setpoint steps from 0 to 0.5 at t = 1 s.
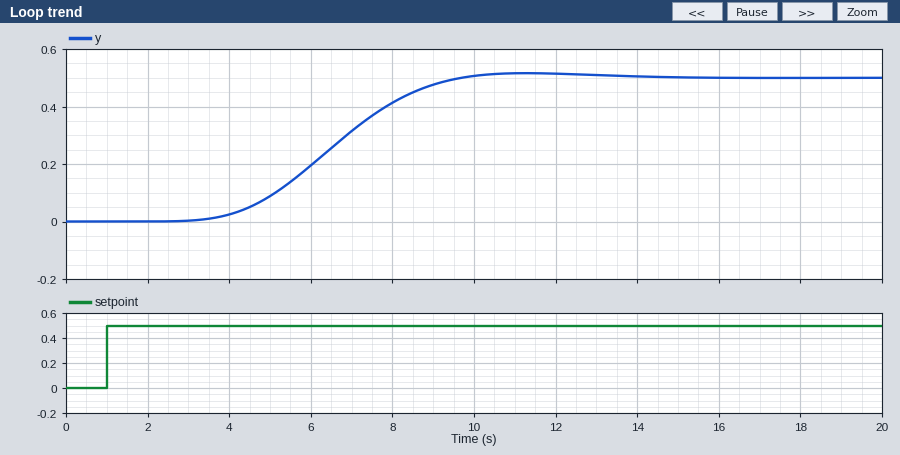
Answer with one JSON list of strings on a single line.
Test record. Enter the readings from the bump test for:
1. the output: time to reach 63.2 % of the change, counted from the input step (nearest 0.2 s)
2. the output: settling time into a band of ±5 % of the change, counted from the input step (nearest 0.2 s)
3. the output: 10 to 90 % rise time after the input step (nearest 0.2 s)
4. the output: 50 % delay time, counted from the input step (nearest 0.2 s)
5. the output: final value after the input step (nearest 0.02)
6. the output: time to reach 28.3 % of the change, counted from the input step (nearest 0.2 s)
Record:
["6.0 s", "8.0 s", "4.0 s", "5.4 s", "0.50", "4.6 s"]
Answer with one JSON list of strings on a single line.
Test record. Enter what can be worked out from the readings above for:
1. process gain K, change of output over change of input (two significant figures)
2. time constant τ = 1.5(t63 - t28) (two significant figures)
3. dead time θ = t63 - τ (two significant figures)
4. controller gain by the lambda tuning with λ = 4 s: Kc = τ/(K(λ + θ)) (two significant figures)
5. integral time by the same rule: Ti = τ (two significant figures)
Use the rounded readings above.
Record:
["1.0", "2.1 s", "3.9 s", "0.27", "2.1 s"]
